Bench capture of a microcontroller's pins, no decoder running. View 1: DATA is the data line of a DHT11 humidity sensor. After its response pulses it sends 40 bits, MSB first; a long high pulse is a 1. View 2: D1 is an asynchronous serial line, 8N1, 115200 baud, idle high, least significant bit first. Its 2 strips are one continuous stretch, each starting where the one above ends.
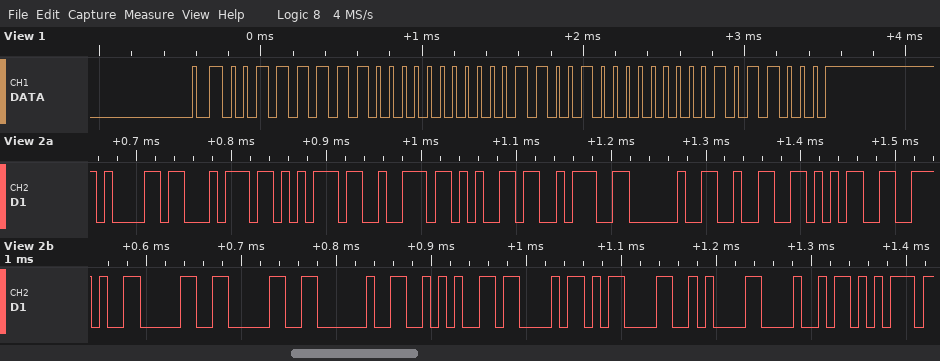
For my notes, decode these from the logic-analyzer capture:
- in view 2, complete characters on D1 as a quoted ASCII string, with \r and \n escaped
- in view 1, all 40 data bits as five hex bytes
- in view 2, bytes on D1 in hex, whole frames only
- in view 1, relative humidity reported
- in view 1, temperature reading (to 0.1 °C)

"ature: 25.00 *C\r\nHu"
3F 00 19 00 58
61 74 75 72 65 3A 20 32 35 2E 30 30 20 2A 43 0D 0A 48 75
63 %
25.0 °C
